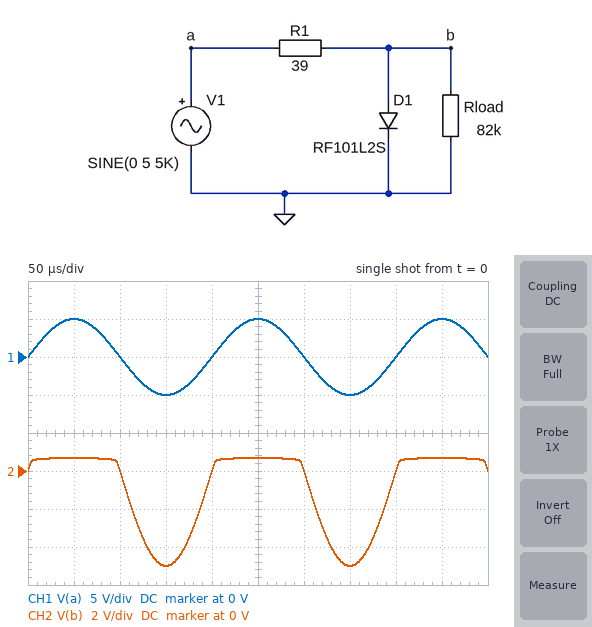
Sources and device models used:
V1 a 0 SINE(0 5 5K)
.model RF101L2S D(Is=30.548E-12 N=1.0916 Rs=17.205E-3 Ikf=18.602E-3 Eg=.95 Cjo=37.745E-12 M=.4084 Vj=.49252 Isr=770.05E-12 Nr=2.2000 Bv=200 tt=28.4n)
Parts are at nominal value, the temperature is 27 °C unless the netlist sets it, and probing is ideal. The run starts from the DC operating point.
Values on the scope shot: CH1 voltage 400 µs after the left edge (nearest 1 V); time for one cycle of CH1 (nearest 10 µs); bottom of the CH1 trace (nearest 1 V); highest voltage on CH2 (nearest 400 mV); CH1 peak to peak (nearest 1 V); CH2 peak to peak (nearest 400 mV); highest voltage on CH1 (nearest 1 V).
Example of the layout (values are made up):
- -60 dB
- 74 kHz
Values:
- 0 V
- 200 µs
- -5 V
- 800 mV
- 10 V
- 5.6 V
- 5 V
